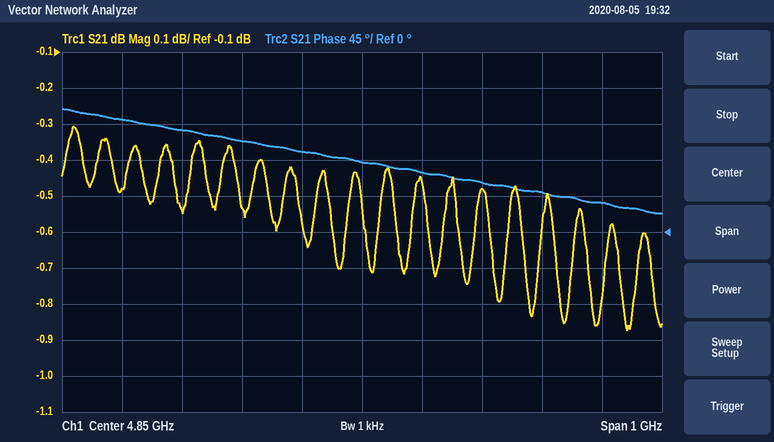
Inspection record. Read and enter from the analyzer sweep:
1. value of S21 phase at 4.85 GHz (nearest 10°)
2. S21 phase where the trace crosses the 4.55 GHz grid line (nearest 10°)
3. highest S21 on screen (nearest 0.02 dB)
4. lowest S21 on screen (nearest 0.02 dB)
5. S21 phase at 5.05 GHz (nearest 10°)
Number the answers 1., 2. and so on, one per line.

1. 90°
2. 130°
3. -0.30 dB
4. -0.88 dB
5. 60°
